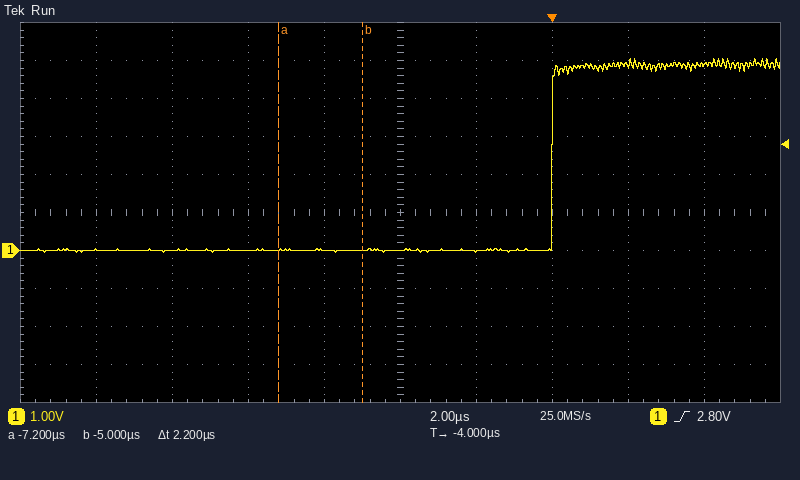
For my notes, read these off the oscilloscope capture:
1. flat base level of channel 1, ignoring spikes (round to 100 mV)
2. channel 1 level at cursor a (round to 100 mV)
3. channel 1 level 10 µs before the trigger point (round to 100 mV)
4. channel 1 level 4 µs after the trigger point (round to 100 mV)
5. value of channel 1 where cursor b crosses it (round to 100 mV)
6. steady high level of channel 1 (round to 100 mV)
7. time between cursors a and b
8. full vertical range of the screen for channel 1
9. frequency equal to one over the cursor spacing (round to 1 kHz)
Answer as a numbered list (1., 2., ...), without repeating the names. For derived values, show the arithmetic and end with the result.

1. 0.0 V
2. 0.0 V
3. 0.0 V
4. 4.9 V
5. 0.0 V
6. 4.9 V
7. 2.2 µs
8. 10 V
9. 1 / 2.2 µs ≈ 455 kHz
